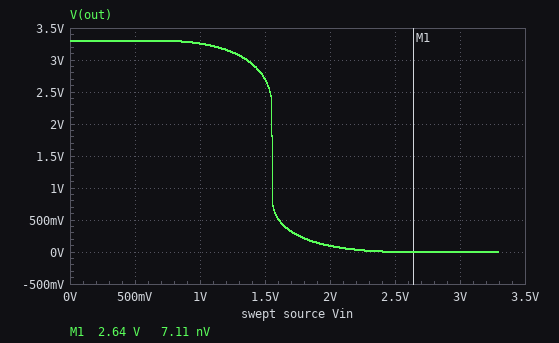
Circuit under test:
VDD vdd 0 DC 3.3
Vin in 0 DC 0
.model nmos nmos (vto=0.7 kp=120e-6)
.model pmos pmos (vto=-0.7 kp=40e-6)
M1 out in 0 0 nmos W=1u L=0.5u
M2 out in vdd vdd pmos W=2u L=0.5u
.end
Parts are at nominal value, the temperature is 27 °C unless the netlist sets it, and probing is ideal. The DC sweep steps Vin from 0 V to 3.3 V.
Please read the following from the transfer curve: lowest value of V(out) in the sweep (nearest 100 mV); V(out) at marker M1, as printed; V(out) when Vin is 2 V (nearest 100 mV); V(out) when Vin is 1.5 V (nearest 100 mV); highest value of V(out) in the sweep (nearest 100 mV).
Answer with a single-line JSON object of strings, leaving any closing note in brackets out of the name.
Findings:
{"lowest value of V(out) in the sweep": "0 V", "V(out) at marker M1, as printed": "7.11 nV", "V(out) when Vin is 2 V": "100 mV", "V(out) when Vin is 1.5 V": "2.7 V", "highest value of V(out) in the sweep": "3.3 V"}
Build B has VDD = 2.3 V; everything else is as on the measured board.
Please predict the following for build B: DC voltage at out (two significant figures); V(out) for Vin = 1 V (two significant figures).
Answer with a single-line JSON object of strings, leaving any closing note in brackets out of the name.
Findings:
{"DC voltage at out": "2.3 V", "V(out) for Vin = 1 V": "2.2 V"}
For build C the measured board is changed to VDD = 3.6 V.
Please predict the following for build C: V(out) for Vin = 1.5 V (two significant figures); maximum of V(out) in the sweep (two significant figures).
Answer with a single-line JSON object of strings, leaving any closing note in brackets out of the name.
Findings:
{"V(out) for Vin = 1.5 V": "3.2 V", "maximum of V(out) in the sweep": "3.6 V"}
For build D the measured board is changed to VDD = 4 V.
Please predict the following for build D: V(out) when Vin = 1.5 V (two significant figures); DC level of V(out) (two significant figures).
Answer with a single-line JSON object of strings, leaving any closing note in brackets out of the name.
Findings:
{"V(out) when Vin = 1.5 V": "3.7 V", "DC level of V(out)": "4.0 V"}
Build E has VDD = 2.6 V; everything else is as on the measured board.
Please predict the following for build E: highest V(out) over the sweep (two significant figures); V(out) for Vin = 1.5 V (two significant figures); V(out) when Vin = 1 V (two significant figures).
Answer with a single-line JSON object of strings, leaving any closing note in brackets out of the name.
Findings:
{"highest V(out) over the sweep": "2.6 V", "V(out) for Vin = 1.5 V": "70 mV", "V(out) when Vin = 1 V": "2.5 V"}
